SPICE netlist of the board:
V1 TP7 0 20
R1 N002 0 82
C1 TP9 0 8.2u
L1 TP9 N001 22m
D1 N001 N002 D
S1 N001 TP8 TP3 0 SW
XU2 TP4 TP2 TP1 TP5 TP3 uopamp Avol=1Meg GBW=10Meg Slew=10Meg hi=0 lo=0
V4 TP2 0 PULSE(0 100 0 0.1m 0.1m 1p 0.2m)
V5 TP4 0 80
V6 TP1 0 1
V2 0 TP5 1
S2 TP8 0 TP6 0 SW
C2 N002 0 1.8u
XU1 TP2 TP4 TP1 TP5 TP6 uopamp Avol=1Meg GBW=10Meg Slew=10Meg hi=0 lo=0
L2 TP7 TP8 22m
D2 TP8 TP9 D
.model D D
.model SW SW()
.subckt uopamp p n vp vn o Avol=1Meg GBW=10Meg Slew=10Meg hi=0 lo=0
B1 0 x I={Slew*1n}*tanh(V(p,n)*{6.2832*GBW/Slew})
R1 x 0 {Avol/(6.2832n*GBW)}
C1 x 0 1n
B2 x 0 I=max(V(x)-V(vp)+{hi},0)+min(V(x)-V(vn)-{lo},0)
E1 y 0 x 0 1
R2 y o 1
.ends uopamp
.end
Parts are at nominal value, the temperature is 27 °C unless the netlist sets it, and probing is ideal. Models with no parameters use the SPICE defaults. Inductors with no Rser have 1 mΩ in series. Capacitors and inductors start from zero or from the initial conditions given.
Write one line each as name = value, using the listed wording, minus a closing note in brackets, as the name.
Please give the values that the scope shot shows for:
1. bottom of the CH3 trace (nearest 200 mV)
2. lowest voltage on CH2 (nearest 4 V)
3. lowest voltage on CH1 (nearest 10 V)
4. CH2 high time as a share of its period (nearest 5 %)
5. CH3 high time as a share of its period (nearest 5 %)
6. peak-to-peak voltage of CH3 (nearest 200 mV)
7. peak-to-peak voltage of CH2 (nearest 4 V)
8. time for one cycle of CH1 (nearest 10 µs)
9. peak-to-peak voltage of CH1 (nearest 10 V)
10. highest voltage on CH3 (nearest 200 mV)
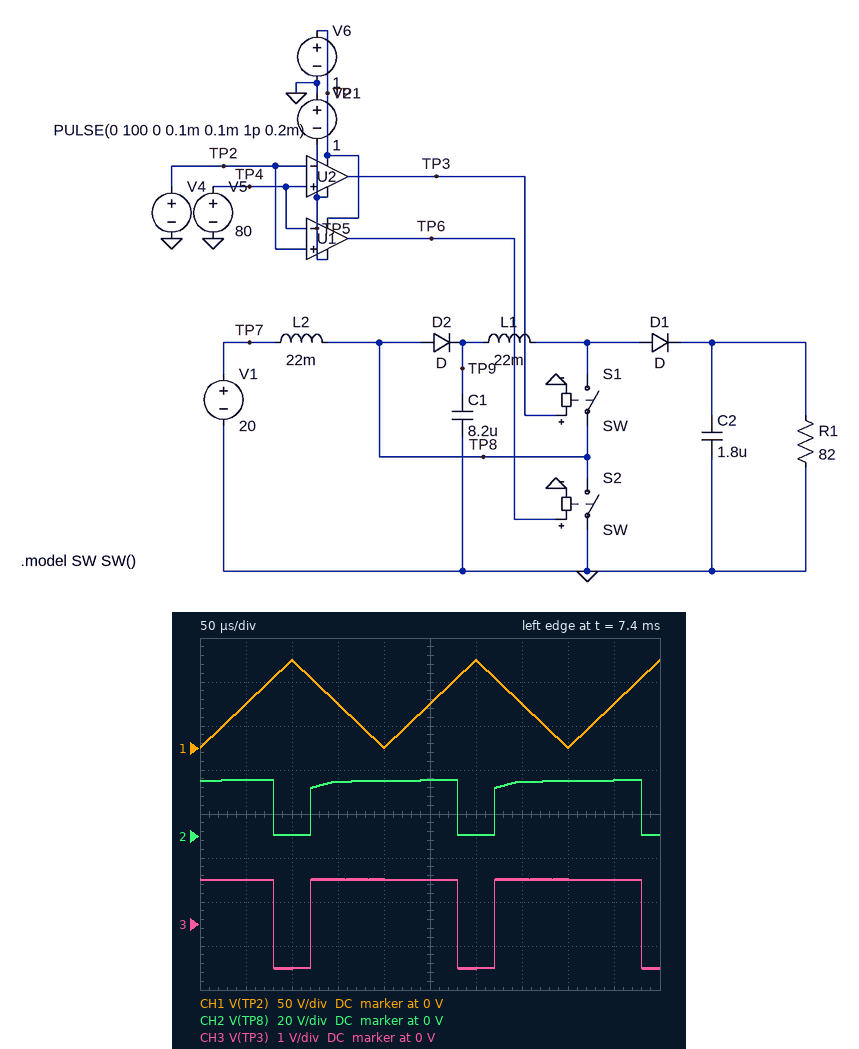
bottom of the CH3 trace = -1.0 V
lowest voltage on CH2 = 0 V
lowest voltage on CH1 = 0 V
CH2 high time as a share of its period = 80 %
CH3 high time as a share of its period = 80 %
peak-to-peak voltage of CH3 = 2.0 V
peak-to-peak voltage of CH2 = 24 V
time for one cycle of CH1 = 200 µs
peak-to-peak voltage of CH1 = 100 V
highest voltage on CH3 = 1.0 V
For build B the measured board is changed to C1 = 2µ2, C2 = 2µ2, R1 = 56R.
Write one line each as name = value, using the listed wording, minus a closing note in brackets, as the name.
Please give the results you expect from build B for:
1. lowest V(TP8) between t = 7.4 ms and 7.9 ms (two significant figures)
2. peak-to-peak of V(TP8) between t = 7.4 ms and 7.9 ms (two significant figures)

lowest V(TP8) between t = 7.4 ms and 7.9 ms = 500 mV
peak-to-peak of V(TP8) between t = 7.4 ms and 7.9 ms = 26 V
